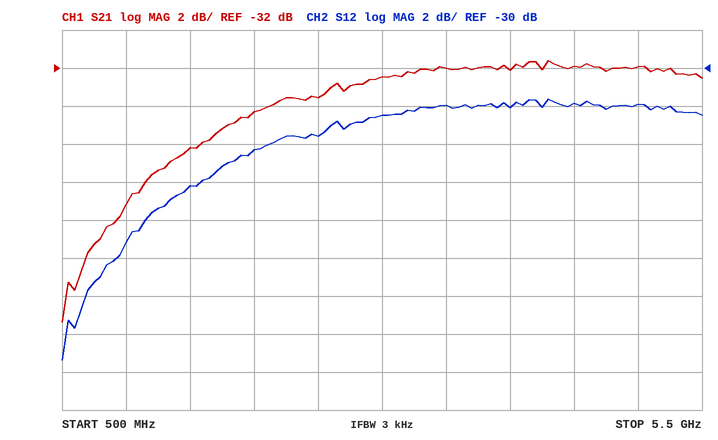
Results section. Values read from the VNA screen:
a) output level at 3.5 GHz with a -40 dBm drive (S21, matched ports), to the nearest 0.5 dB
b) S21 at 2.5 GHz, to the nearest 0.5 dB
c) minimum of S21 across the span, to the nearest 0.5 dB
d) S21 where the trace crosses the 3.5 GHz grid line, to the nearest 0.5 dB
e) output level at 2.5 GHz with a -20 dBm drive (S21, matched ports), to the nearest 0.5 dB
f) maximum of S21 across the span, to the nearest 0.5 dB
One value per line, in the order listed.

-72.0 dBm
-33.5 dB
-45.5 dB
-32.0 dB
-53.5 dBm
-31.5 dB
